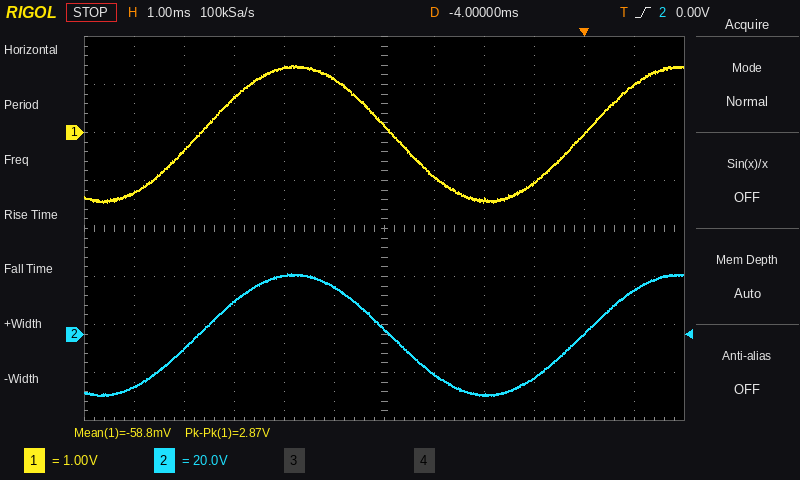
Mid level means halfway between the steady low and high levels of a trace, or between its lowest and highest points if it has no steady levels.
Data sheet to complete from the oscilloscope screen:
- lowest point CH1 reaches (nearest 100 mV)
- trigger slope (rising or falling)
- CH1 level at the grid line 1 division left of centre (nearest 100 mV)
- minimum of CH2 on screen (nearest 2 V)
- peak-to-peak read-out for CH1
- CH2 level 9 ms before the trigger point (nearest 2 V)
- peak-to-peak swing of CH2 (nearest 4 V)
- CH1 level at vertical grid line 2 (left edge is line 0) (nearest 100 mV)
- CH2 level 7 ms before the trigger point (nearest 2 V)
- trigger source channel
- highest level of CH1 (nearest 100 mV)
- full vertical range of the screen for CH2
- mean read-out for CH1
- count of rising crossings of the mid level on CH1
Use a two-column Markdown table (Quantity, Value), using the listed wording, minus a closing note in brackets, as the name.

| Quantity | Value |
|---|---|
| lowest point CH1 reaches | -1.5 V |
| trigger slope | rising |
| CH1 level at the grid line 1 division left of centre | 1.1 V |
| minimum of CH2 on screen | -26 V |
| peak-to-peak read-out for CH1 | 2.87 V |
| CH2 level 9 ms before the trigger point | -22 V |
| peak-to-peak swing of CH2 | 52 V |
| CH1 level at vertical grid line 2 (left edge is line 0) | -400 mV |
| CH2 level 7 ms before the trigger point | 14 V |
| trigger source channel | CH2 |
| highest level of CH1 | 1.4 V |
| full vertical range of the screen for CH2 | 160 V |
| mean read-out for CH1 | -58.8 mV |
| count of rising crossings of the mid level on CH1 | 2 |
